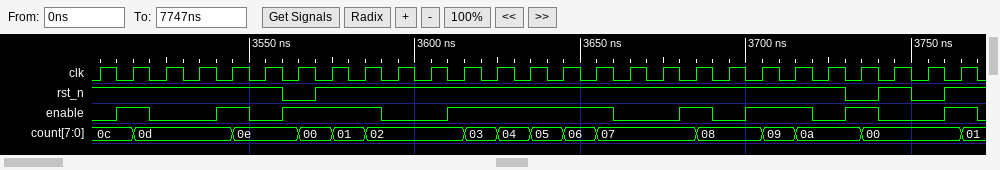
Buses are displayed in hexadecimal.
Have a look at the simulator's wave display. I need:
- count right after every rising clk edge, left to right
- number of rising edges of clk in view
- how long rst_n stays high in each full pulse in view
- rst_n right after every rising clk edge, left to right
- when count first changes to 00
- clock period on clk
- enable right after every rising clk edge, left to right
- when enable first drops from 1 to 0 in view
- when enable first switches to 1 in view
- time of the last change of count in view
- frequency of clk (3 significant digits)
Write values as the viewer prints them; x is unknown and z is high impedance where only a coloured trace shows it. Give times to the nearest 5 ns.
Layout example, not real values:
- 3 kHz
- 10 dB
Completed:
- 0c, 0d, 0d, 0d, 0e, 0e, 00, 01, 02, 02, 02, 03, 04, 05, 06, 07, 07, 07, 08, 08, 09, 0a, 0a, 00, 00, 00, 01
- 27
- 160 ns, 10 ns
- 1 1 1 1 1 1 0 1 1 1 1 1 1 1 1 1 1 1 1 1 1 1 1 0 1 0 1
- 3565 ns
- 10 ns
- 0 1 0 0 1 0 1 1 1 0 0 1 1 1 1 1 0 0 1 0 1 1 0 1 0 0 1
- 3520 ns
- 3510 ns
- 3765 ns
- 100 MHz
